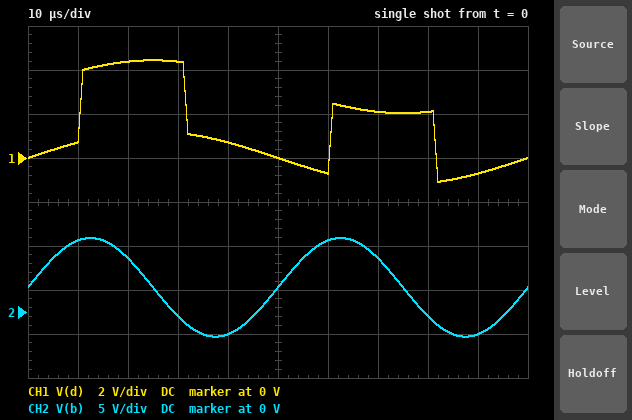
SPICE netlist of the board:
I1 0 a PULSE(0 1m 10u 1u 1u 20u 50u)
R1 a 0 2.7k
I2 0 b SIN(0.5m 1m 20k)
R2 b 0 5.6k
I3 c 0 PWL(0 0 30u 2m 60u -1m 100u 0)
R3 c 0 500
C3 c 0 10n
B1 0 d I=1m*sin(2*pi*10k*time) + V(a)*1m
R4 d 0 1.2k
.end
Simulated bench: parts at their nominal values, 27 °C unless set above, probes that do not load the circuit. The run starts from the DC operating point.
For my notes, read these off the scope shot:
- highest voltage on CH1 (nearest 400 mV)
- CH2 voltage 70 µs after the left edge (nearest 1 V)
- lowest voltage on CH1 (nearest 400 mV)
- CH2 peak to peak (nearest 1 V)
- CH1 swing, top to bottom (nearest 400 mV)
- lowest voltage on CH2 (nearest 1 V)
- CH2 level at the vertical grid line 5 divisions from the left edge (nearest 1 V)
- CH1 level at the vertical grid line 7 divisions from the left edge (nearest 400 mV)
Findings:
4.4 V
6 V
-1.2 V
11 V
5.6 V
-3 V
3 V
2.0 V
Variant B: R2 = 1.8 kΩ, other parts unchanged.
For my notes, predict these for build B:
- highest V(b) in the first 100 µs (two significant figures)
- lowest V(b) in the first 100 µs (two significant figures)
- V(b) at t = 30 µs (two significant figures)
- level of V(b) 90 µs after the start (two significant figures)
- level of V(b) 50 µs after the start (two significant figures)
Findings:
2.7 V
-900 mV
-160 mV
-810 mV
900 mV
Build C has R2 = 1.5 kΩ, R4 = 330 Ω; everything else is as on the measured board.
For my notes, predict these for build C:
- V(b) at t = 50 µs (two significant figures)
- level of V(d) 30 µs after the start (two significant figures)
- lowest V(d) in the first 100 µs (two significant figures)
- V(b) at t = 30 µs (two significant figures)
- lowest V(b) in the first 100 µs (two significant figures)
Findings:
750 mV
1.2 V
-300 mV
-130 mV
-750 mV
